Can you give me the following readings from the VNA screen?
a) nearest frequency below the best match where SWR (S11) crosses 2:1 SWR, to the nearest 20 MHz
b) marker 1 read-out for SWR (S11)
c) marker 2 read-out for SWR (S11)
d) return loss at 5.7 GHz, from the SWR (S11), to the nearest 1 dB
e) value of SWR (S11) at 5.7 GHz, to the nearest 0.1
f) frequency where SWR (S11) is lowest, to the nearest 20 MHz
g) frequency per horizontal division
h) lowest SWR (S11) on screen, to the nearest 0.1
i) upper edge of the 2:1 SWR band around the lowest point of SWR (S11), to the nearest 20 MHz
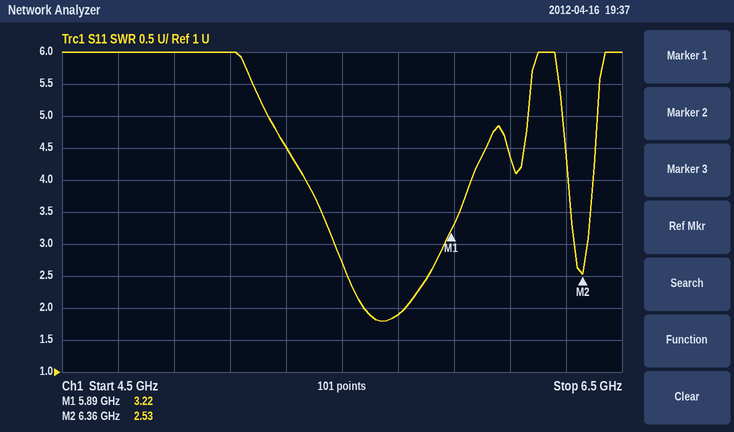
5.58 GHz
3.22
2.53
10 dB
1.9
5.64 GHz
200 MHz
1.8
5.72 GHz
